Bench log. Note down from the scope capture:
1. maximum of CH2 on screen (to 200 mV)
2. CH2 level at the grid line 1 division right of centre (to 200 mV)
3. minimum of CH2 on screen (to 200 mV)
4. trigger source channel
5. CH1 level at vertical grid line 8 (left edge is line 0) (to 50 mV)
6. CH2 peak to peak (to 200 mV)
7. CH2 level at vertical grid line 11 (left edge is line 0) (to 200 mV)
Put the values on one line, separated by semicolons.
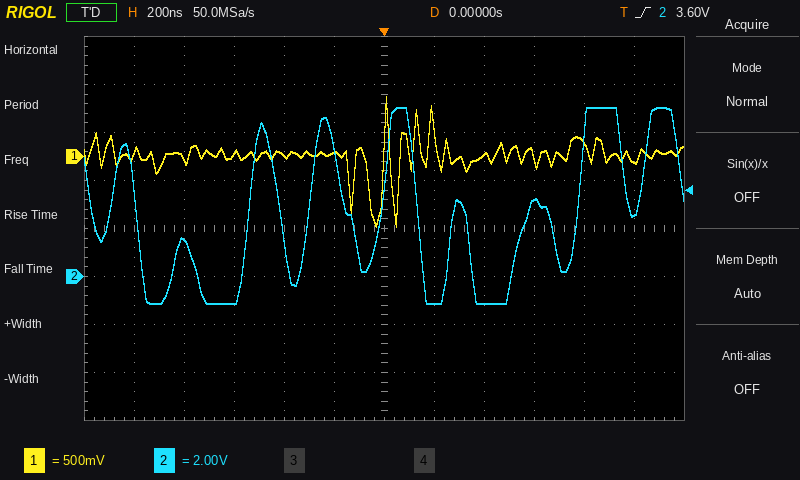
7.0 V; -1.2 V; -1.2 V; CH2; 0 mV; 8.2 V; 2.6 V
